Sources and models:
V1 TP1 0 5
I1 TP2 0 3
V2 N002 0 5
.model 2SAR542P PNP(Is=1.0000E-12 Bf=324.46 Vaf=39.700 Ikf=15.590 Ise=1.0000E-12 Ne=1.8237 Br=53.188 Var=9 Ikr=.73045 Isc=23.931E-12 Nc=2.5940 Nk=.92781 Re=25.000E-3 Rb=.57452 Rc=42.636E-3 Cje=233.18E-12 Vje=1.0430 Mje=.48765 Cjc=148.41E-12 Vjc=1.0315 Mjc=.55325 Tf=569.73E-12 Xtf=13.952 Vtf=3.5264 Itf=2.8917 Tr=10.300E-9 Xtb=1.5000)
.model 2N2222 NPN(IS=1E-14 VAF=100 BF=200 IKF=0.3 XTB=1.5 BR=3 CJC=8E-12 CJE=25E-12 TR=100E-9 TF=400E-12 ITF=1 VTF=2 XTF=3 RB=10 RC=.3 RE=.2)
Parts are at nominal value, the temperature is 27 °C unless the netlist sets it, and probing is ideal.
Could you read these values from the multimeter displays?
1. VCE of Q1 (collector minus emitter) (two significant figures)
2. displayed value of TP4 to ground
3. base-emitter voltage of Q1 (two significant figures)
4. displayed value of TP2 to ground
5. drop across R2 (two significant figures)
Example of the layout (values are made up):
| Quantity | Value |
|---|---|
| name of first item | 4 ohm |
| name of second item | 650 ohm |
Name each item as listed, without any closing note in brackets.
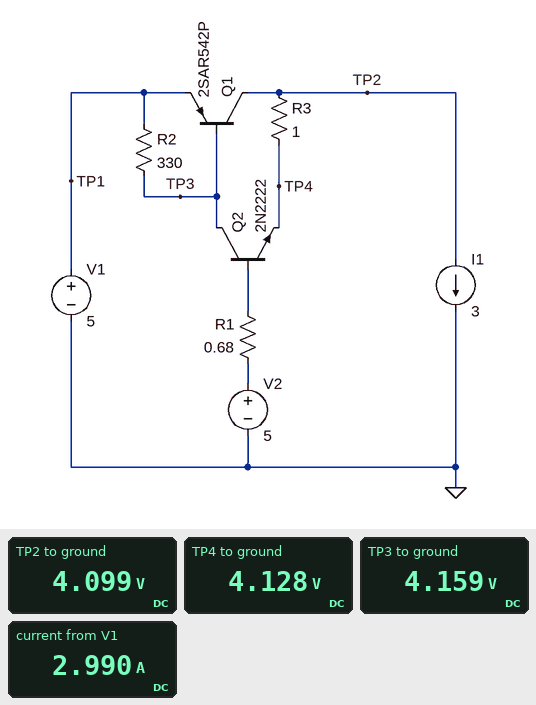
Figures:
| Quantity | Value |
|---|---|
| VCE of Q1 (collector minus emitter) | -900 mV |
| displayed value of TP4 to ground | 4.128 V |
| base-emitter voltage of Q1 | -840 mV |
| displayed value of TP2 to ground | 4.099 V |
| drop across R2 | 840 mV |
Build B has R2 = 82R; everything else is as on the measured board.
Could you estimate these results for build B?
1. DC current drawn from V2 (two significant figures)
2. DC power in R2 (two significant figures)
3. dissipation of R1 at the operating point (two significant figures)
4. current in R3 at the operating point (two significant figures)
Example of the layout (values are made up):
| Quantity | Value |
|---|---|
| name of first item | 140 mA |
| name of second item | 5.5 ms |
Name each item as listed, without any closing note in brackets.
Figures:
| Quantity | Value |
|---|---|
| DC current drawn from V2 | 10 mA |
| DC power in R2 | 8.6 mW |
| dissipation of R1 at the operating point | 68 µW |
| current in R3 at the operating point | 36 mA |
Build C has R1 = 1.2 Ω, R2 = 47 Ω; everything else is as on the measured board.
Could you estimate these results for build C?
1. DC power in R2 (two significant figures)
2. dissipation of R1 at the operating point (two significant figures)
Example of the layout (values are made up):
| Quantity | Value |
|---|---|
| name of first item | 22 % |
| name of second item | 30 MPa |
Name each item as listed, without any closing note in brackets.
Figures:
| Quantity | Value |
|---|---|
| DC power in R2 | 15 mW |
| dissipation of R1 at the operating point | 110 µW |
